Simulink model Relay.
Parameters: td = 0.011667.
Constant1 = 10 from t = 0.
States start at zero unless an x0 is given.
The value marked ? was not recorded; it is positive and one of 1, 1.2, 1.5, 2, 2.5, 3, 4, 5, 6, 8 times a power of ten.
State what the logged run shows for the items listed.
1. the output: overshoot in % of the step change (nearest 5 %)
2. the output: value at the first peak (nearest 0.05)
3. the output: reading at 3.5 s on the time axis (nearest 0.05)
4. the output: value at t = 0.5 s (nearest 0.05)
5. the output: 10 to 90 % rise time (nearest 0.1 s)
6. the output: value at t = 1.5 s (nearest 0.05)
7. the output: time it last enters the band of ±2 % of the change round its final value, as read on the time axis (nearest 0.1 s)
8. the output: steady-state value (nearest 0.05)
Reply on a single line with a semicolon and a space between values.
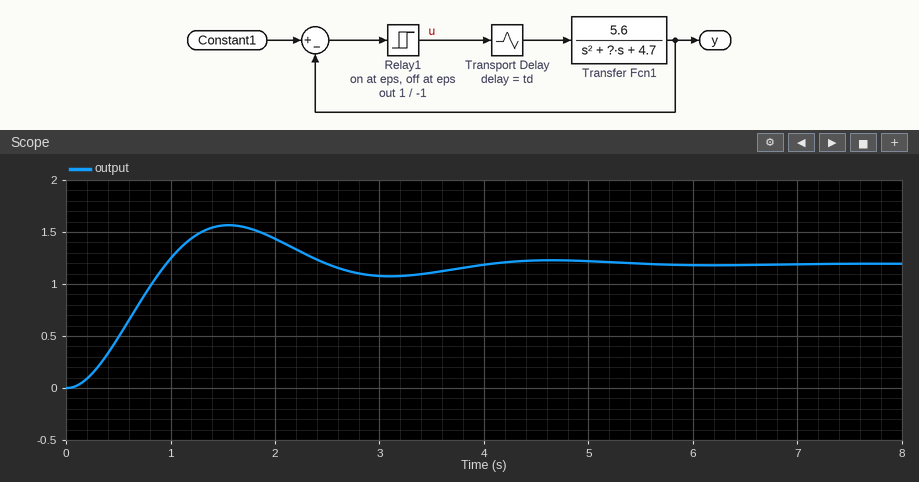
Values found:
30 %; 1.55; 1.10; 0.50; 0.6 s; 1.55; 5.1 s; 1.20
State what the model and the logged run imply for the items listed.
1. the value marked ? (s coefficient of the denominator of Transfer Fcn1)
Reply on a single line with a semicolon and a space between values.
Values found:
1.5
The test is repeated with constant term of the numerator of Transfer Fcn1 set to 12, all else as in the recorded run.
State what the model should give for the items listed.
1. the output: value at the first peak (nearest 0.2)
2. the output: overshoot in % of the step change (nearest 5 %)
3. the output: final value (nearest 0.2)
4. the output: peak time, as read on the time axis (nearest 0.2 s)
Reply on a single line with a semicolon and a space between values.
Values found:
3.4; 30 %; 2.6; 1.6 s
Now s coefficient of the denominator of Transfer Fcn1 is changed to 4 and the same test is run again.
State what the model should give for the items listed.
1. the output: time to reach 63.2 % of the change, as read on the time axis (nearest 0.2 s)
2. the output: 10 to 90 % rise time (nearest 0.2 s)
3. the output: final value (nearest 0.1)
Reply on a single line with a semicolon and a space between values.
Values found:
1.0 s; 1.4 s; 1.2
